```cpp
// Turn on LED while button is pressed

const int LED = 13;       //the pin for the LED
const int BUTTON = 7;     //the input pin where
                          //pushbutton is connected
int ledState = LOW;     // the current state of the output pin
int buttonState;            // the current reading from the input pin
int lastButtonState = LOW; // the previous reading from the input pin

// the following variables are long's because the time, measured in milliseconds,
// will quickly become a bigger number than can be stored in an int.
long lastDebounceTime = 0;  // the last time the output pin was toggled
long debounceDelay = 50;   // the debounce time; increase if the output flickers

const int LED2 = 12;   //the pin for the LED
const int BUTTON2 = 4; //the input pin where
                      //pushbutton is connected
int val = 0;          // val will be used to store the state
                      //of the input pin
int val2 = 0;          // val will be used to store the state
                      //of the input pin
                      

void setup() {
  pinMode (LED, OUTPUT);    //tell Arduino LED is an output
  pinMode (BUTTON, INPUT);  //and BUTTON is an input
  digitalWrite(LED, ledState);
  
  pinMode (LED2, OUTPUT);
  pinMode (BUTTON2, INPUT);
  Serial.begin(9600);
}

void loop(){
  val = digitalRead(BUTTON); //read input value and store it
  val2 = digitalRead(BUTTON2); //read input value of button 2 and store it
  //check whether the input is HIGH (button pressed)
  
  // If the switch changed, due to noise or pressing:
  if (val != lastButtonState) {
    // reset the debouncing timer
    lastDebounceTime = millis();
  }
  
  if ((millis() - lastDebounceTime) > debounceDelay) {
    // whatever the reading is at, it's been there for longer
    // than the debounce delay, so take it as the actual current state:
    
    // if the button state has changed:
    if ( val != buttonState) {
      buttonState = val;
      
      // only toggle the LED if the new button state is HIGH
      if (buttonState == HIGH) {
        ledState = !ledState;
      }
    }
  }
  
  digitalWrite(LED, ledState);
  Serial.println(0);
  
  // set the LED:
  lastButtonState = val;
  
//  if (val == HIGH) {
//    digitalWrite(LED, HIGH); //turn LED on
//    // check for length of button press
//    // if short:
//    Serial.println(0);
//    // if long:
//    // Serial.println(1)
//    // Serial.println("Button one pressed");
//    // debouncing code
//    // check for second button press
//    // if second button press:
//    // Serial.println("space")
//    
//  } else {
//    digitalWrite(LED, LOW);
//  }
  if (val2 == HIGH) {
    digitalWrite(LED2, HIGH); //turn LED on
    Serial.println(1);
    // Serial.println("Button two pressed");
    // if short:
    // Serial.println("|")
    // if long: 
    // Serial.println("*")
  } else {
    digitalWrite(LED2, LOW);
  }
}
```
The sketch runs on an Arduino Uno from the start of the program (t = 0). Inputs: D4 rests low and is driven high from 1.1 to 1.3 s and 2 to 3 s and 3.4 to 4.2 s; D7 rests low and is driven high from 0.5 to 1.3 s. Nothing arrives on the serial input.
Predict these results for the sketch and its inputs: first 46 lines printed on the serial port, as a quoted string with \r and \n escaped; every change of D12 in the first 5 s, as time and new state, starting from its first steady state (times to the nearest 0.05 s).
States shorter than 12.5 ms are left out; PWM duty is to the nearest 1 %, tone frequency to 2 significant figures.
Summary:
"0\r\n0\r\n0\r\n0\r\n0\r\n0\r\n0\r\n0\r\n0\r\n0\r\n0\r\n0\r\n0\r\n0\r\n0\r\n0\r\n0\r\n0\r\n0\r\n0\r\n0\r\n0\r\n0\r\n0\r\n0\r\n0\r\n0\r\n0\r\n0\r\n0\r\n0\r\n0\r\n0\r\n0\r\n0\r\n0\r\n0\r\n0\r\n0\r\n0\r\n0\r\n0\r\n0\r\n0\r\n0\r\n0\r\n"
0 s low; 1.1 s high; 1.3 s low; 2 s high; 3 s low; 3.4 s high; 4.2 s low
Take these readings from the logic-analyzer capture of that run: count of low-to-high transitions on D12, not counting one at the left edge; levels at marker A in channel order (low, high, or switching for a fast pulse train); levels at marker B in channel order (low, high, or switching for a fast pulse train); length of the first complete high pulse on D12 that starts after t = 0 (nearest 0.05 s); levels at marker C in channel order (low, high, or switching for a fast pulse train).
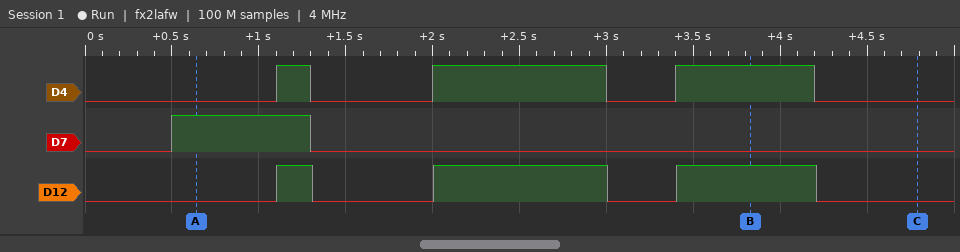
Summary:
3
D4 low, D7 high, D12 low
D4 high, D7 low, D12 high
0.20 s
D4 low, D7 low, D12 low
